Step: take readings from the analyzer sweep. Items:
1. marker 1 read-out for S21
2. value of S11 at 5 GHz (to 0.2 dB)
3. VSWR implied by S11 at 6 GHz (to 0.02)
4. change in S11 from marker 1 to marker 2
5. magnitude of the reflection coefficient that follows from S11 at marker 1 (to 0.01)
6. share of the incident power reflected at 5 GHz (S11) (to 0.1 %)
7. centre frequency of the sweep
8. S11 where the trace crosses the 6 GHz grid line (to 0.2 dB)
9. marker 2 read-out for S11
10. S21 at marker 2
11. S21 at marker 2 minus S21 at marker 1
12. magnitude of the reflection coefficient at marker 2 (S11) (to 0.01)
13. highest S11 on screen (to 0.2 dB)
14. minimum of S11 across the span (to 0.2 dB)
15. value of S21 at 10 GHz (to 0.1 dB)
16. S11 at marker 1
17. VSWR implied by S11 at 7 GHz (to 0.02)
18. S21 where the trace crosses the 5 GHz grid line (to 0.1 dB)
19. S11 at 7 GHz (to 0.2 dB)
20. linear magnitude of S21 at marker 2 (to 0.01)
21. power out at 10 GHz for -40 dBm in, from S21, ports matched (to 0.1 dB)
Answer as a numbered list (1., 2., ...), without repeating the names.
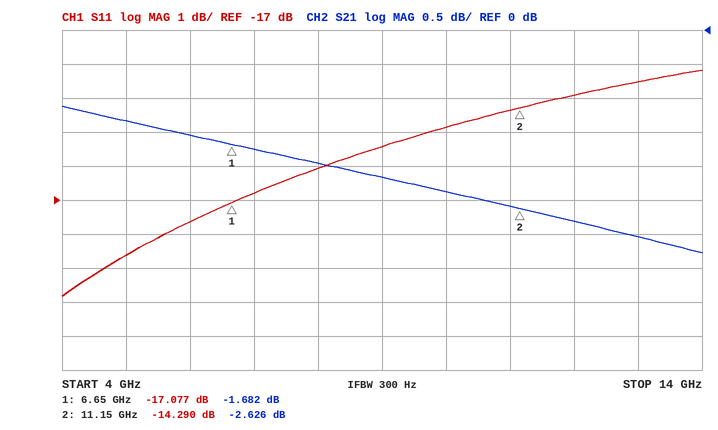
1. -1.682 dB
2. -18.6 dB
3. 1.30
4. 2.787 dB
5. 0.14
6. 1.4 %
7. 9 GHz
8. -17.6 dB
9. -14.290 dB
10. -2.626 dB
11. -0.944 dB
12. 0.19
13. -13.2 dB
14. -19.8 dB
15. -2.4 dB
16. -17.077 dB
17. 1.34
18. -1.3 dB
19. -16.8 dB
20. 0.74
21. -42.4 dBm
